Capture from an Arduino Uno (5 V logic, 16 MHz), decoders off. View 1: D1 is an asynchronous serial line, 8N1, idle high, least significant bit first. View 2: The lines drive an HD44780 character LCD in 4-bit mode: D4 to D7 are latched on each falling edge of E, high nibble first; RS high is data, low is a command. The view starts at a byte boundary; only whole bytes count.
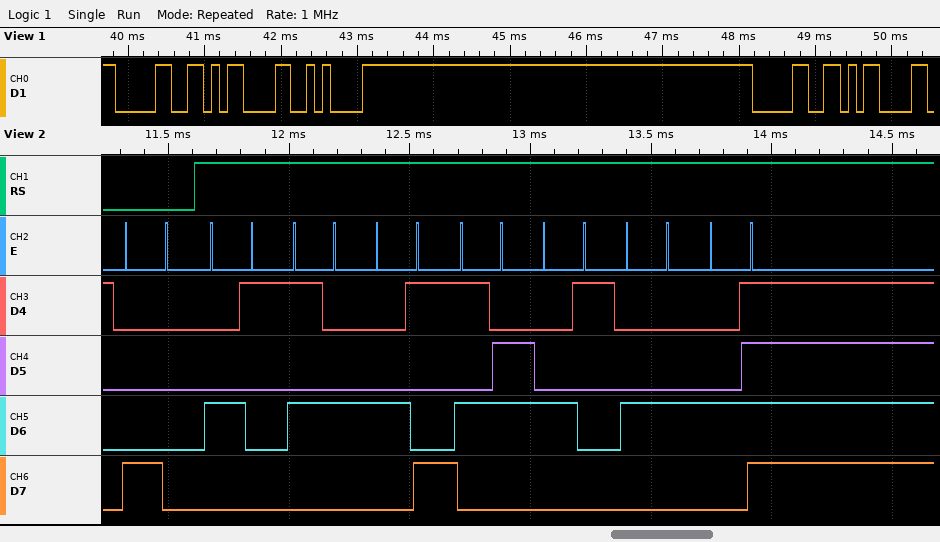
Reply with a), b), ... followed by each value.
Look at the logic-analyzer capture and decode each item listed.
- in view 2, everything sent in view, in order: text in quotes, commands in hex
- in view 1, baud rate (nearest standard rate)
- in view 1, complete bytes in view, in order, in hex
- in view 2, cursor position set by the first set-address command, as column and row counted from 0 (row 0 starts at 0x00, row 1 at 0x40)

a) 0x80 "ATIVADO"
b) 9600 baud
c) 30 0D 0A 30 0D
d) column 0, row 0
